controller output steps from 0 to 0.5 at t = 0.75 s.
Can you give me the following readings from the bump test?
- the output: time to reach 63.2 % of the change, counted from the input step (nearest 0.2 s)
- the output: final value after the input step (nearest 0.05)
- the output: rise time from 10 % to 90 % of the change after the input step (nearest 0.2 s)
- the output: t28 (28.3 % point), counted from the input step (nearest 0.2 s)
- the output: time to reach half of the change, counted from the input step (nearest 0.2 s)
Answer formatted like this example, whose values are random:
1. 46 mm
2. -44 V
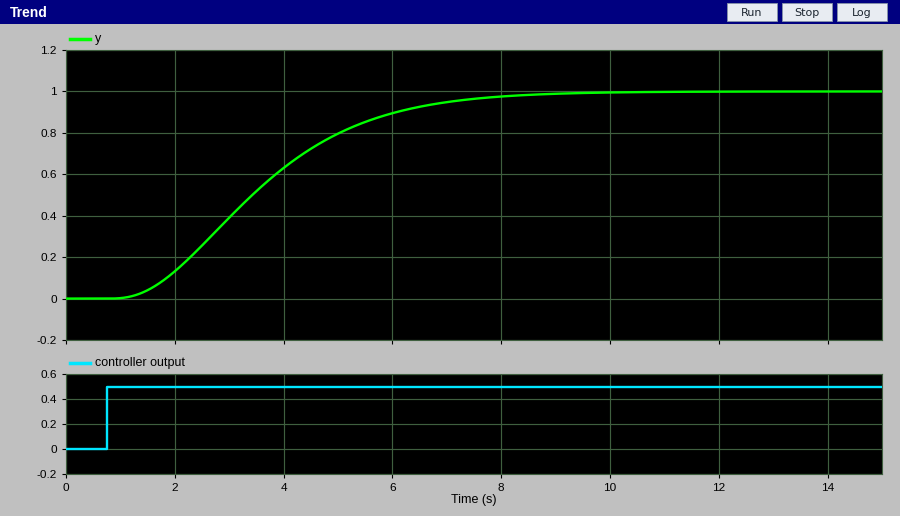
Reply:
1. 3.2 s
2. 1.00
3. 4.2 s
4. 1.8 s
5. 2.6 s
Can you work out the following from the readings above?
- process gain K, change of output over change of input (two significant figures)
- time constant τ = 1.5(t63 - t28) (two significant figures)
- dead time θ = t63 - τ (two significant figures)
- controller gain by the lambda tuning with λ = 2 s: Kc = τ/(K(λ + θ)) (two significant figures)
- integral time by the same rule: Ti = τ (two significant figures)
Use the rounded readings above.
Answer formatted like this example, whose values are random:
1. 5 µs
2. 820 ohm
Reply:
1. 2.0
2. 2.1 s
3. 1.1 s
4. 0.34
5. 2.1 s
